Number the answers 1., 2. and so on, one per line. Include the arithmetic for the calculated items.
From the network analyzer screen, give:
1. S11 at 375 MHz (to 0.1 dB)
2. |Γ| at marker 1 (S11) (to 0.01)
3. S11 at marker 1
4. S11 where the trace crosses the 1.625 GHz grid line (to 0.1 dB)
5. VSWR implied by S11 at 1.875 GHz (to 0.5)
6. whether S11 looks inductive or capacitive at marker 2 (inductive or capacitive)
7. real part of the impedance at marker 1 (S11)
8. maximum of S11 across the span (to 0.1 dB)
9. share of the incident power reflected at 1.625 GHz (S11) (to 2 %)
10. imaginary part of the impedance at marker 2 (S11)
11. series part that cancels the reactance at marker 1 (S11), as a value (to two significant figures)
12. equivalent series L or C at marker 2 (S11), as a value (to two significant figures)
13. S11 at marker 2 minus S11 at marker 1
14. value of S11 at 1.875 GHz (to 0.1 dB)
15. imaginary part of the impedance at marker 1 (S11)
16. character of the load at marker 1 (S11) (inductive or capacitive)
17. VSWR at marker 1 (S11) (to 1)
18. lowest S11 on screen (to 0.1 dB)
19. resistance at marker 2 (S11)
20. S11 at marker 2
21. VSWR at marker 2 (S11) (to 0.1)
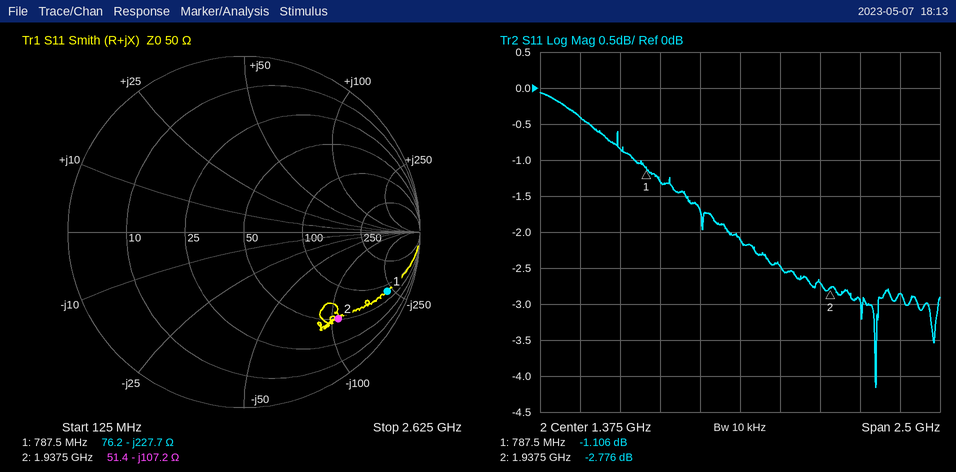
1. -0.4 dB
2. 0.88
3. -1.106 dB
4. -2.5 dB
5. |Γ| = 10^(-2.7/20) = 0.7328; VSWR = (1 + 0.7328)/(1 − 0.7328) ≈ 6.5
6. capacitive
7. 76.2 Ω
8. -0.1 dB
9. 10^(-2.5/10) ≈ 56 %
10. -107.2 Ω
11. L = 227.7 Ω/(2π × 787.5 MHz) ≈ 46 nH
12. C = 1/(2π × 1.9375 GHz × 107.2 Ω) ≈ 766 fF, so 770 fF to two significant figures
13. -2.776 − (-1.106) = -1.670 dB
14. -2.7 dB
15. -227.7 Ω
16. capacitive
17. (1 + 0.8804)/(1 − 0.8804) ≈ 16
18. -4.2 dB
19. 51.4 Ω
20. -2.776 dB
21. 6.3
